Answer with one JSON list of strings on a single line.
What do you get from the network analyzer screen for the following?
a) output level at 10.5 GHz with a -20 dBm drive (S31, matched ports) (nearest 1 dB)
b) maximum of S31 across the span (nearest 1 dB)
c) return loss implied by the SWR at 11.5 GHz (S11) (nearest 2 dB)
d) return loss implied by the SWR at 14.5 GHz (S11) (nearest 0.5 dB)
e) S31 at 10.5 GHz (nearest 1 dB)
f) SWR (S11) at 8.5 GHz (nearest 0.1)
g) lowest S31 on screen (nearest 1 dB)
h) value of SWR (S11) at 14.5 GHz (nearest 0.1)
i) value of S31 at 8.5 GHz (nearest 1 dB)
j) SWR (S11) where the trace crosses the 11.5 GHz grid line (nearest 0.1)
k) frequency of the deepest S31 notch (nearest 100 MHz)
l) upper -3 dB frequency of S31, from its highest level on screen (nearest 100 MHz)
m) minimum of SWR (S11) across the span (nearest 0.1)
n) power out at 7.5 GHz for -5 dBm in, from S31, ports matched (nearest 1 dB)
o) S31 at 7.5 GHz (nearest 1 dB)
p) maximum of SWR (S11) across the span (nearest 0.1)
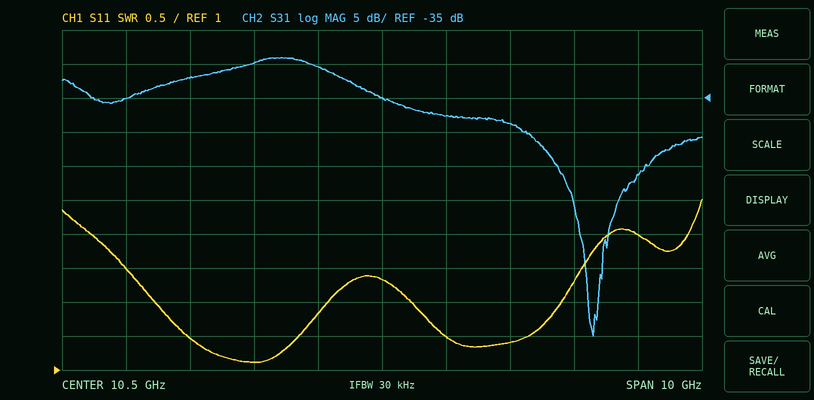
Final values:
["-55 dBm", "-29 dB", "14 dB", "6.0 dB", "-35 dB", "1.1", "-70 dB", "3.0", "-30 dB", "1.5", "13.8 GHz", "9.9 GHz", "1.1", "-37 dBm", "-32 dB", "3.5"]
